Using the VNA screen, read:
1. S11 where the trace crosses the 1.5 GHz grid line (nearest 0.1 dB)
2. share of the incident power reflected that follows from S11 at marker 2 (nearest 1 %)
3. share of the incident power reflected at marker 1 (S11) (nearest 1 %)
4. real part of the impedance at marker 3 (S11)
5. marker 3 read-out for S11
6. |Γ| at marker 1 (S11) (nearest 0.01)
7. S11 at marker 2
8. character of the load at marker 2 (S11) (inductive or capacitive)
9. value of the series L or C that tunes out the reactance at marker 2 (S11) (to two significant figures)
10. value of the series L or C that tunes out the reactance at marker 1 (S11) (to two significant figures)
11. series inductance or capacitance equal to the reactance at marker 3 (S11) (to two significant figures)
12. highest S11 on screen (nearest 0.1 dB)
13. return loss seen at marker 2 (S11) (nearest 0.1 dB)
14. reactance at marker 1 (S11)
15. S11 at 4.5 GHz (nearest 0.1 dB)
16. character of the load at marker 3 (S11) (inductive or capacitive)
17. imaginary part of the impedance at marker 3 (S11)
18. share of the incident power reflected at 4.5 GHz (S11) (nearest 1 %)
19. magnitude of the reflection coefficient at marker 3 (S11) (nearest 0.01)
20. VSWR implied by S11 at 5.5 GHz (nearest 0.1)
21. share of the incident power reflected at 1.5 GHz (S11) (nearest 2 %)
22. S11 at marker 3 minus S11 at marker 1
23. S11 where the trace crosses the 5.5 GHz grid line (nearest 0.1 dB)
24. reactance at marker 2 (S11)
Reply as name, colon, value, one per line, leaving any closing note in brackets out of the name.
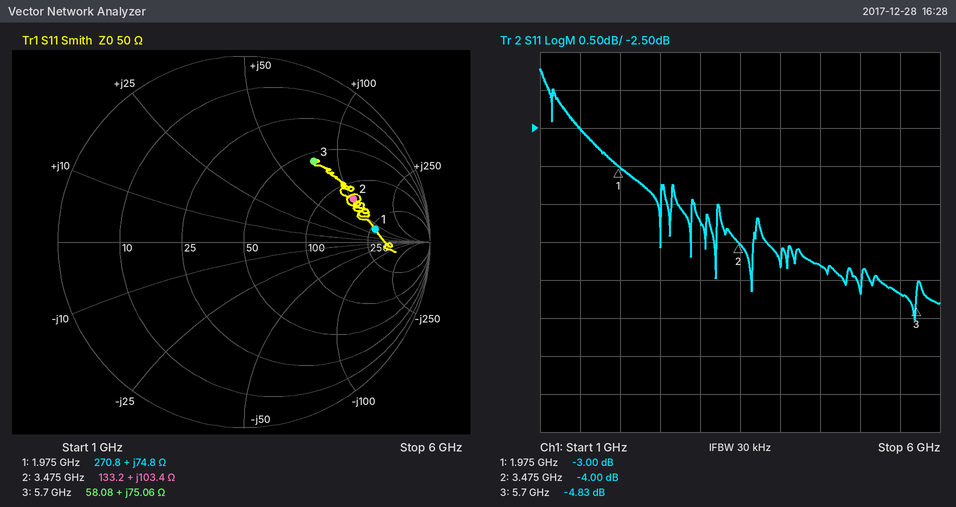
S11 where the trace crosses the 1.5 GHz grid line: -2.5 dB
share of the incident power reflected that follows from S11 at marker 2: 40 %
share of the incident power reflected at marker 1 (S11): 50 %
real part of the impedance at marker 3: 58.08 Ω
marker 3 read-out for S11: -4.83 dB
|Γ| at marker 1 (S11): 0.71
S11 at marker 2: -4.00 dB
character of the load at marker 2 (S11): inductive
value of the series L or C that tunes out the reactance at marker 2 (S11): 440 fF
value of the series L or C that tunes out the reactance at marker 1 (S11): 1.1 pF
series inductance or capacitance equal to the reactance at marker 3 (S11): 2.1 nH
highest S11 on screen: -1.7 dB
return loss seen at marker 2 (S11): 4.0 dB
reactance at marker 1: +74.8 Ω
S11 at 4.5 GHz: -4.3 dB
character of the load at marker 3 (S11): inductive
imaginary part of the impedance at marker 3: +75.06 Ω
share of the incident power reflected at 4.5 GHz (S11): 37 %
magnitude of the reflection coefficient at marker 3 (S11): 0.57
VSWR implied by S11 at 5.5 GHz: 3.8
share of the incident power reflected at 1.5 GHz (S11): 56 %
S11 at marker 3 minus S11 at marker 1: -1.83 dB
S11 where the trace crosses the 5.5 GHz grid line: -4.7 dB
reactance at marker 2: +103.4 Ω
